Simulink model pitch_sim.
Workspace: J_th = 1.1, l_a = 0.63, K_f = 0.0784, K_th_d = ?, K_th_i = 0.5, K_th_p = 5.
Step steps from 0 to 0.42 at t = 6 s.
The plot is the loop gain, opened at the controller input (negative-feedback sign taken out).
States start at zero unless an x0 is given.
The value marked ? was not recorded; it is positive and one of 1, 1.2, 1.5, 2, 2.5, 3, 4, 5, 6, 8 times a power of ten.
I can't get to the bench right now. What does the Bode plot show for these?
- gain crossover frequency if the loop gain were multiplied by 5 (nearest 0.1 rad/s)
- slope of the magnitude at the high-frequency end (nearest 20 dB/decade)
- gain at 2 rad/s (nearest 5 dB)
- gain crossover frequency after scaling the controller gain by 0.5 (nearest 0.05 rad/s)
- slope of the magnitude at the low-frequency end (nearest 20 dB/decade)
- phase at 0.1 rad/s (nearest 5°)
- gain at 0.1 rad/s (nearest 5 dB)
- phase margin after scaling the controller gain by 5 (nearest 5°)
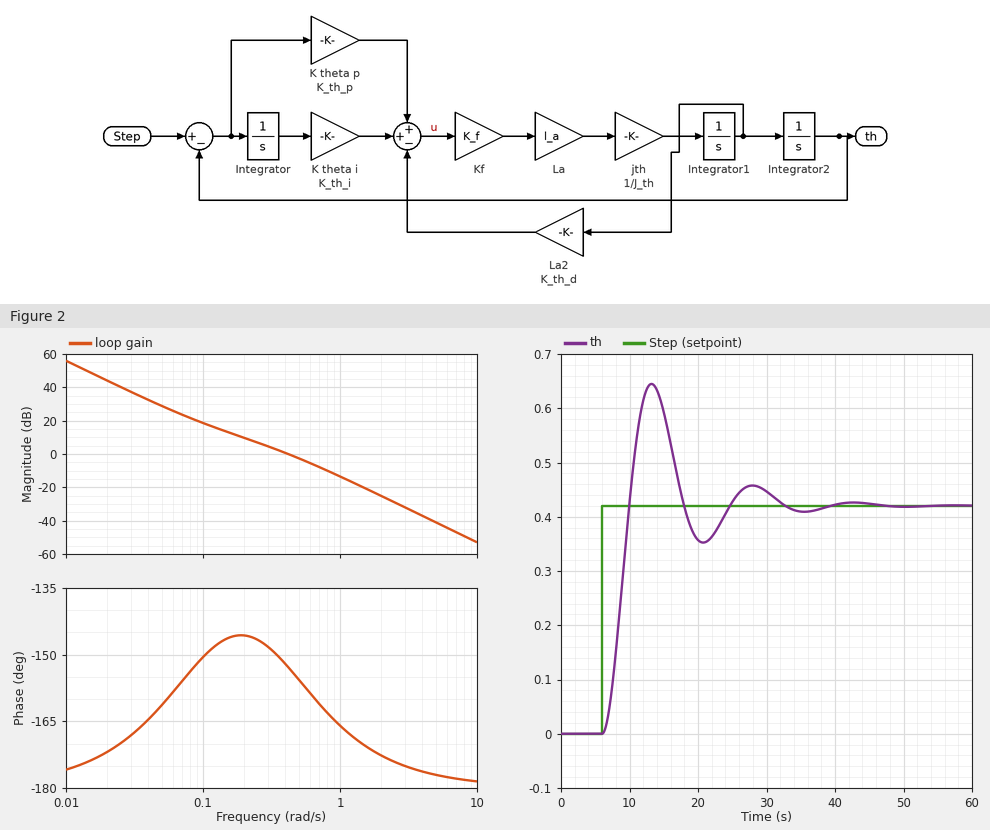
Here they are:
1.0 rad/s
-40 dB/decade
-25 dB
0.25 rad/s
-40 dB/decade
-150°
20 dB
15°
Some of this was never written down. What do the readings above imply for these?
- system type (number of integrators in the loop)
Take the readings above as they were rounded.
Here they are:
2
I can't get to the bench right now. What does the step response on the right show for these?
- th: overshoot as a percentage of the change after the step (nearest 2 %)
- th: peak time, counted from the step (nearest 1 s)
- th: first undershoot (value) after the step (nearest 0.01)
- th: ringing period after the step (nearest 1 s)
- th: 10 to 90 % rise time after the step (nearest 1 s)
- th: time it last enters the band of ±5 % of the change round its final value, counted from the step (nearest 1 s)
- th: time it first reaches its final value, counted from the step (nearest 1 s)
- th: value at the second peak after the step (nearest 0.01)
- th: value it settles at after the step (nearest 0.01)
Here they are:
54 %
7 s
0.35
15 s
3 s
25 s
4 s
0.46
0.42
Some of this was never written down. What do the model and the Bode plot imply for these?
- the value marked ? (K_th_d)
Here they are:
8
